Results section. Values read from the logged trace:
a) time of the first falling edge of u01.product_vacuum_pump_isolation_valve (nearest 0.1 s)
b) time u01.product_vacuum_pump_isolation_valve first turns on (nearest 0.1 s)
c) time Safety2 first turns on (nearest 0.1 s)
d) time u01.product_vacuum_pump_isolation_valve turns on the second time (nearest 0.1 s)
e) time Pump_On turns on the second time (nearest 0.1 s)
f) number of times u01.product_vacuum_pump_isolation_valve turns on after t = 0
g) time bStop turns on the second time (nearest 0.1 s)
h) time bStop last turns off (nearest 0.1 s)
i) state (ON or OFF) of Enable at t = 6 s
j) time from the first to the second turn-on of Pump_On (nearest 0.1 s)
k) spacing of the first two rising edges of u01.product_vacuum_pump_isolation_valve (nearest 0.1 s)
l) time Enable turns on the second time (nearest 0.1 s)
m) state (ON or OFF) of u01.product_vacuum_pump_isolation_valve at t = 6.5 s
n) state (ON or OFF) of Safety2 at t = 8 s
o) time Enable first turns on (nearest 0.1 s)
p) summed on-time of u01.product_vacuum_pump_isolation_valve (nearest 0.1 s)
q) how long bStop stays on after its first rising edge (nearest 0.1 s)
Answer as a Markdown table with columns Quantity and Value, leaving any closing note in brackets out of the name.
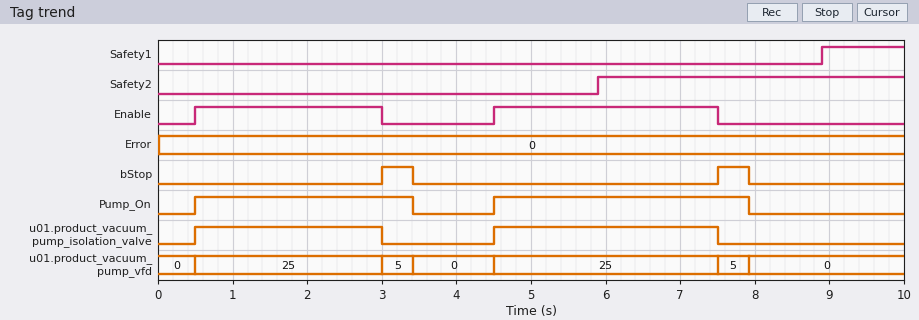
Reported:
| Quantity | Value |
|---|---|
| time of the first falling edge of u01.product_vacuum_pump_isolation_valve | 3.0 s |
| time u01.product_vacuum_pump_isolation_valve first turns on | 0.5 s |
| time Safety2 first turns on | 5.9 s |
| time u01.product_vacuum_pump_isolation_valve turns on the second time | 4.5 s |
| time Pump_On turns on the second time | 4.5 s |
| number of times u01.product_vacuum_pump_isolation_valve turns on after t = 0 | 2 |
| time bStop turns on the second time | 7.5 s |
| time bStop last turns off | 7.9 s |
| state (ON or OFF) of Enable at t = 6 s | ON |
| time from the first to the second turn-on of Pump_On | 4.0 s |
| spacing of the first two rising edges of u01.product_vacuum_pump_isolation_valve | 4.0 s |
| time Enable turns on the second time | 4.5 s |
| state (ON or OFF) of u01.product_vacuum_pump_isolation_valve at t = 6.5 s | ON |
| state (ON or OFF) of Safety2 at t = 8 s | ON |
| time Enable first turns on | 0.5 s |
| summed on-time of u01.product_vacuum_pump_isolation_valve | 5.5 s |
| how long bStop stays on after its first rising edge | 0.4 s |
